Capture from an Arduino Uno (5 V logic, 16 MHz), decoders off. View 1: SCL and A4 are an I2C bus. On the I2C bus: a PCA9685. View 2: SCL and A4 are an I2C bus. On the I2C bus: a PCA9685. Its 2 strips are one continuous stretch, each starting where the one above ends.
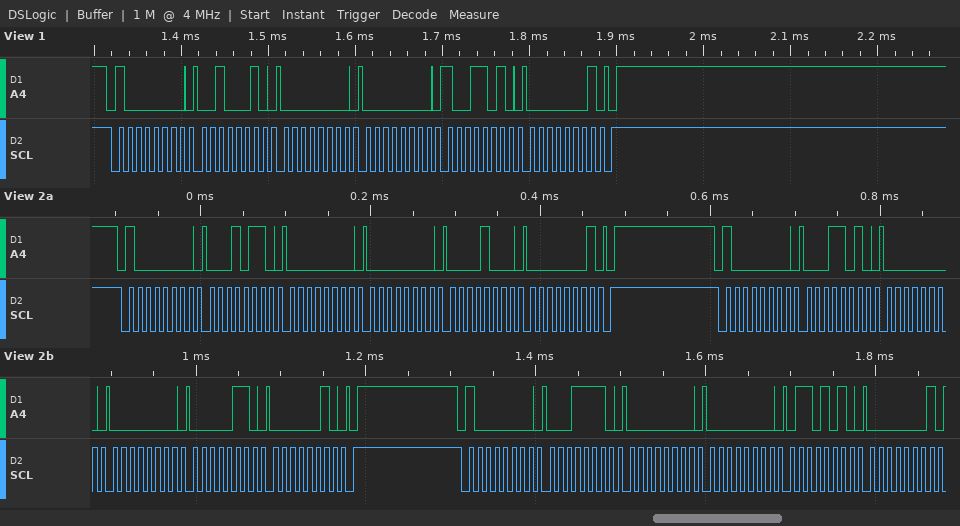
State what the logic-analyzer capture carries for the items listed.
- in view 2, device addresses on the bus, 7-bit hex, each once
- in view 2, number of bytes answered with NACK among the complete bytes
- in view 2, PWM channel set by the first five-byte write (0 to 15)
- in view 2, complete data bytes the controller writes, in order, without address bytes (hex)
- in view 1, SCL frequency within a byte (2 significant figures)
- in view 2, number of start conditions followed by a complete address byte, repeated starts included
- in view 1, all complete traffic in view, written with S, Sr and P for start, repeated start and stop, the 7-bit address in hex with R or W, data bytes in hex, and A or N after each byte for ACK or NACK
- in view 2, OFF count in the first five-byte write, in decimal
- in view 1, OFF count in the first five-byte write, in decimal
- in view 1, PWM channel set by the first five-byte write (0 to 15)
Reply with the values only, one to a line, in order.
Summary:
0x40
0
4
16 00 00 08 01 1A 00 00 06 02 1E 00 00 6A 01
100 kHz
3
S 40W A 22 A 00 A 00 A 9A A 01 A P
264
410
7
